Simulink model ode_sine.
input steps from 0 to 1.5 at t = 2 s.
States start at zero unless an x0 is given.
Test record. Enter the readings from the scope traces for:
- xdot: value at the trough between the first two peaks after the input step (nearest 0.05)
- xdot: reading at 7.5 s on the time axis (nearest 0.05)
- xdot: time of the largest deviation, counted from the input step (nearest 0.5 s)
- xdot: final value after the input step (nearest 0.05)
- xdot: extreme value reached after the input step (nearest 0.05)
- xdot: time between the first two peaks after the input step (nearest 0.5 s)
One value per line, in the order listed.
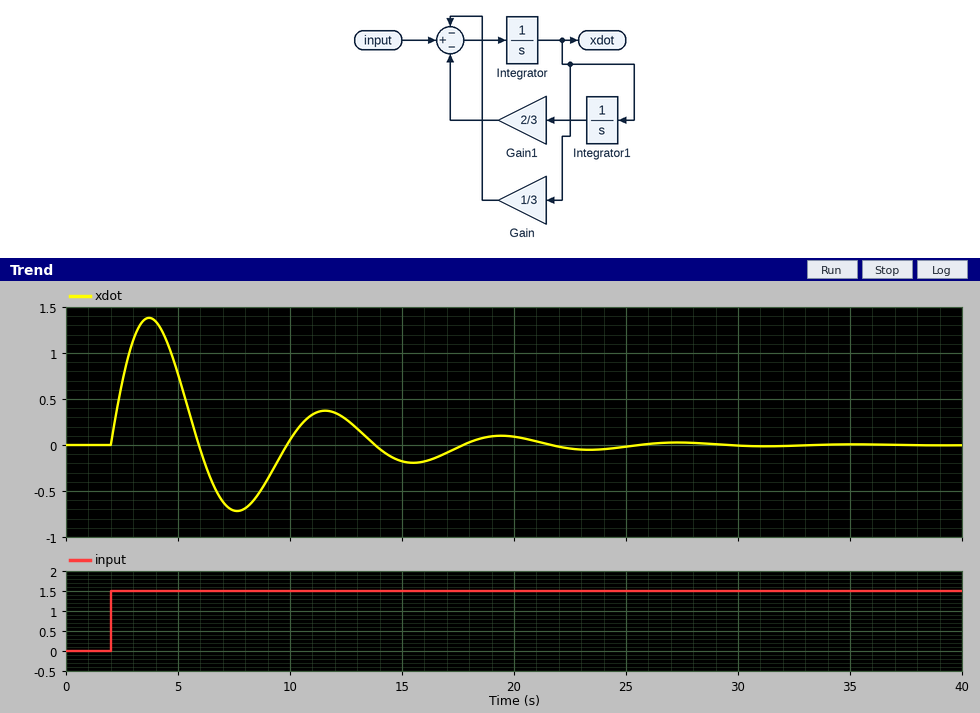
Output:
-0.70
-0.70
1.5 s
0.00
1.40
8.0 s
